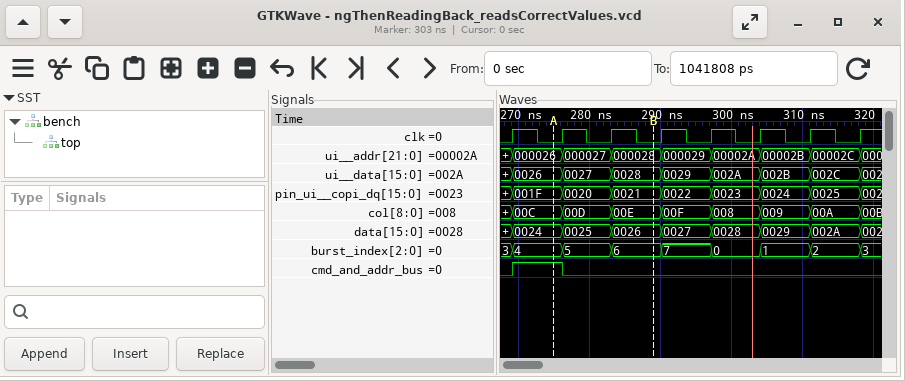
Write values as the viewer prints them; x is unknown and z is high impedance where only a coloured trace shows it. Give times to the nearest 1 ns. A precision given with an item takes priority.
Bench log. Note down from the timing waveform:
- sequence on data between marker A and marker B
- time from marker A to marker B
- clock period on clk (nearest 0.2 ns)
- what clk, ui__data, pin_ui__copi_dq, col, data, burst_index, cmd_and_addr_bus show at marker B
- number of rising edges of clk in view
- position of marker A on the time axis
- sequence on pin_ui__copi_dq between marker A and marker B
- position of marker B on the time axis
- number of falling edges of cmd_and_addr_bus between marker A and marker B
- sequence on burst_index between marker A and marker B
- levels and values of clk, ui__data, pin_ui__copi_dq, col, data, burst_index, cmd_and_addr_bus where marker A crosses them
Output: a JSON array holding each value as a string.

["0024, 0025, 0026", "14 ns", "7 ns", "clk=0, ui__data=0028, pin_ui__copi_dq=0021, col=00E, data=0026, burst_index=6, cmd_and_addr_bus=0", "8", "275 ns", "001F, 0020, 0021", "289 ns", "1", "4, 5, 6", "clk=0, ui__data=0026, pin_ui__copi_dq=001F, col=00C, data=0024, burst_index=4, cmd_and_addr_bus=1"]
